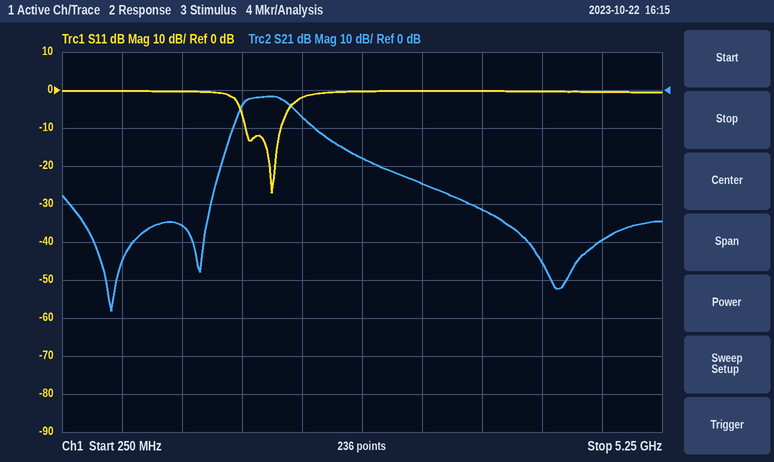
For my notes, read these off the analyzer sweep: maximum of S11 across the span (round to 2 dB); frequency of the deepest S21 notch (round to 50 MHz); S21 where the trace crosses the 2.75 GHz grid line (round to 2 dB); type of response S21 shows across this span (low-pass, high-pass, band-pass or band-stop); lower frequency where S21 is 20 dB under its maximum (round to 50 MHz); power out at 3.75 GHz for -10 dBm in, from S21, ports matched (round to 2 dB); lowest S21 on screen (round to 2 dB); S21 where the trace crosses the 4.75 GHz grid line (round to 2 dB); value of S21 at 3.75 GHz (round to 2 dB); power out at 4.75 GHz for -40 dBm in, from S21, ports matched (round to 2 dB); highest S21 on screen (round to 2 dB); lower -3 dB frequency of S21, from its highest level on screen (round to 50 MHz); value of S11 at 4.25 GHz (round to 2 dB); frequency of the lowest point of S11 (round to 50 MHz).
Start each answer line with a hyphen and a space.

- 0 dB
- 650 MHz
- -18 dB
- band-pass
- 1.55 GHz
- -42 dBm
- -58 dB
- -40 dB
- -32 dB
- -80 dBm
- -2 dB
- 1.75 GHz
- 0 dB
- 2.00 GHz
